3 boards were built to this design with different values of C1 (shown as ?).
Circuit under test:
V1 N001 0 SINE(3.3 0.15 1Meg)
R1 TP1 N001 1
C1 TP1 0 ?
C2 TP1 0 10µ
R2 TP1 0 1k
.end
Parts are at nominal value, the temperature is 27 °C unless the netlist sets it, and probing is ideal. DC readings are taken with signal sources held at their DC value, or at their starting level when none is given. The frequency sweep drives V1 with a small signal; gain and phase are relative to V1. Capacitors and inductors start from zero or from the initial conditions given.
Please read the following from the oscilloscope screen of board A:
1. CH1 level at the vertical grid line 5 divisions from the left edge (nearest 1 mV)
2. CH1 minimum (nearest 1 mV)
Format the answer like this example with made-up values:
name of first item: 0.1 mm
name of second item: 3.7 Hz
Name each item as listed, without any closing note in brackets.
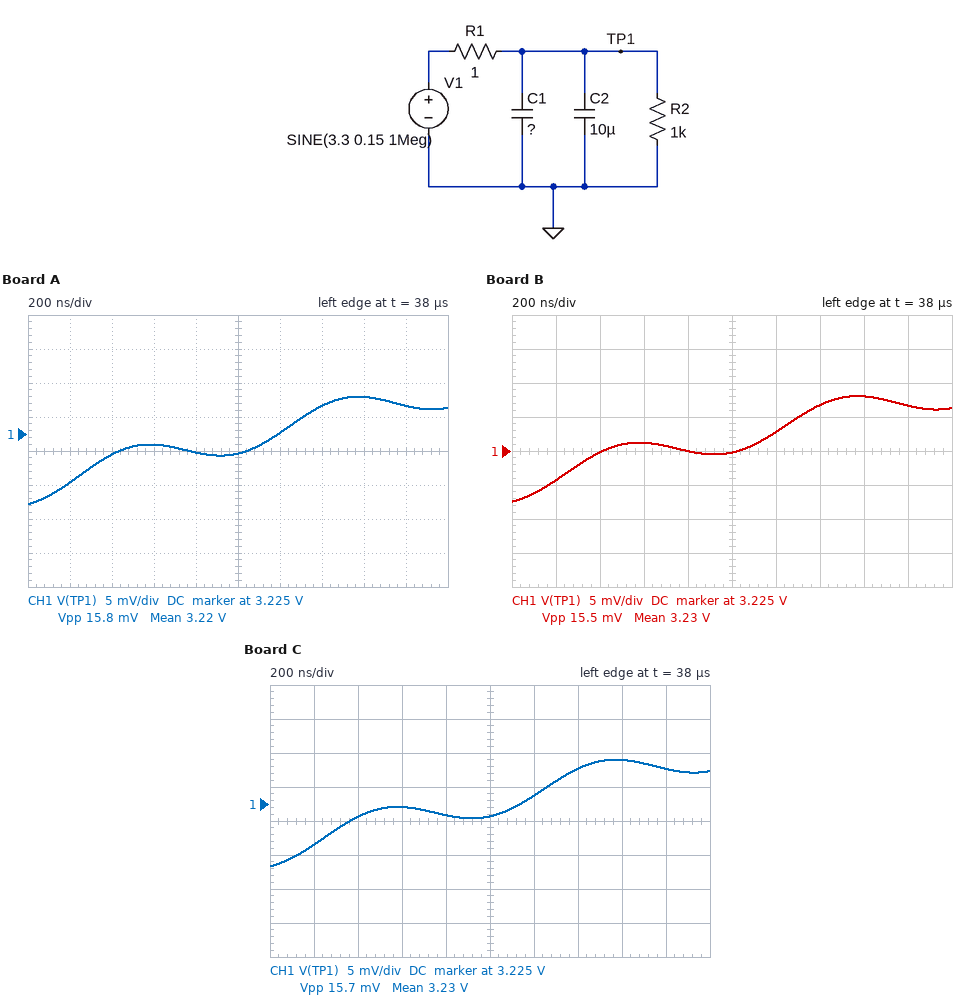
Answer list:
CH1 level at the vertical grid line 5 divisions from the left edge: 3.222 V
CH1 minimum: 3.215 V
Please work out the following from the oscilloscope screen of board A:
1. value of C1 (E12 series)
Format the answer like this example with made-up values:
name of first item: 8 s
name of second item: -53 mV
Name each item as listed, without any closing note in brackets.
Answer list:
value of C1: 220 nF
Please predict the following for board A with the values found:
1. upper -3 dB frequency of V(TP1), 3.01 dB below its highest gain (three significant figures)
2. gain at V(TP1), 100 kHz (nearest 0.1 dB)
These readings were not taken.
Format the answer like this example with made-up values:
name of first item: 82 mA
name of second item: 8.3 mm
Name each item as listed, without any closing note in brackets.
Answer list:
upper -3 dB frequency of V(TP1), 3.01 dB below its highest gain: 15.6 kHz
gain at V(TP1), 100 kHz: -16.3 dB
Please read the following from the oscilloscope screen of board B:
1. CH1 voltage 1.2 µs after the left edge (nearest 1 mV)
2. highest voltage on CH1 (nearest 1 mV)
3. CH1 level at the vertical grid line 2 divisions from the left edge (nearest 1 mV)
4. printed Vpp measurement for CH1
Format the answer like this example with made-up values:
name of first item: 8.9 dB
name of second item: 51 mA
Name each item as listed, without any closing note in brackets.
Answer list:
CH1 voltage 1.2 µs after the left edge: 3.228 V
highest voltage on CH1: 3.233 V
CH1 level at the vertical grid line 2 divisions from the left edge: 3.225 V
printed Vpp measurement for CH1: 15.5 mV
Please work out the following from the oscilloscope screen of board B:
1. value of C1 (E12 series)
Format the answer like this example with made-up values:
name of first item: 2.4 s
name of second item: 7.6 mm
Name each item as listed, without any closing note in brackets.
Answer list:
value of C1: 120 nF
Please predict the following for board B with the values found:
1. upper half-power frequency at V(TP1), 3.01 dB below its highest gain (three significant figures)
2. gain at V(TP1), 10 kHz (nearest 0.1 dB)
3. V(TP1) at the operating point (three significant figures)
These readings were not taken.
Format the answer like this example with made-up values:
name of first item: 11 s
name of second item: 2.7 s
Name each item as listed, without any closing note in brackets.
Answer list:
upper half-power frequency at V(TP1), 3.01 dB below its highest gain: 15.7 kHz
gain at V(TP1), 10 kHz: -1.5 dB
V(TP1) at the operating point: 3.30 V
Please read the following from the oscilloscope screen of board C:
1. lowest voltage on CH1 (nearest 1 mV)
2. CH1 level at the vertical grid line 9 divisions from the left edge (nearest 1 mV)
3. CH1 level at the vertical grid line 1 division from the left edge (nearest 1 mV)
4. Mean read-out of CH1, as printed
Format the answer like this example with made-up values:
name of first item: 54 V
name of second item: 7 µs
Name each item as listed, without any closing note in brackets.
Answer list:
lowest voltage on CH1: 3.216 V
CH1 level at the vertical grid line 9 divisions from the left edge: 3.230 V
CH1 level at the vertical grid line 1 division from the left edge: 3.219 V
Mean read-out of CH1, as printed: 3.23 V
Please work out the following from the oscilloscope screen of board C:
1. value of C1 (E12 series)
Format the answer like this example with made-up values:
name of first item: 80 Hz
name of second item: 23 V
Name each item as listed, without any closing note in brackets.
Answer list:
value of C1: 180 nF
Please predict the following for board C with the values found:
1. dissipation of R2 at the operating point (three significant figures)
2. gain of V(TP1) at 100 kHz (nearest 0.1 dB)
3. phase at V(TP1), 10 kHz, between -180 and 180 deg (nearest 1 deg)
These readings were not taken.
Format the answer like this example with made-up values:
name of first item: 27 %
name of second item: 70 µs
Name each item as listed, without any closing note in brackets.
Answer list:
dissipation of R2 at the operating point: 10.9 mW
gain of V(TP1) at 100 kHz: -16.2 dB
phase at V(TP1), 10 kHz, between -180 and 180 deg: -33 deg
